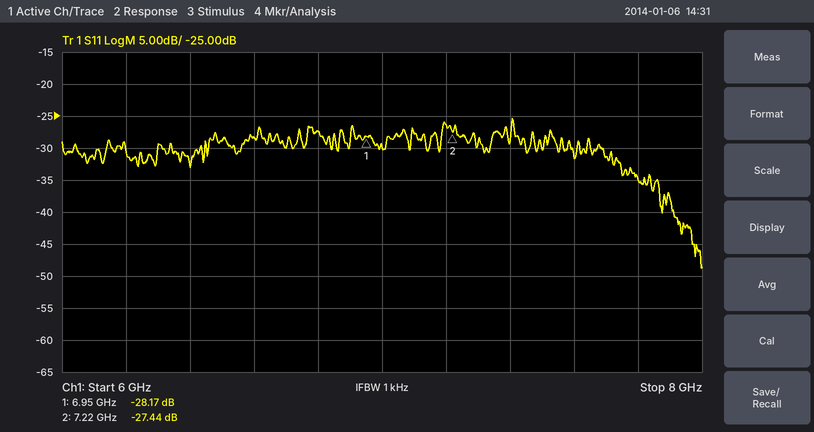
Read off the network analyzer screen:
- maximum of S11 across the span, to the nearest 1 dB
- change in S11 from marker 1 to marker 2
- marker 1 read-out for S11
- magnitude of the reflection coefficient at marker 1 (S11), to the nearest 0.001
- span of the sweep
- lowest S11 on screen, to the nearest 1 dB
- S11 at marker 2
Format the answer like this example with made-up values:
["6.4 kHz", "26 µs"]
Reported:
["-25 dB", "0.73 dB", "-28.17 dB", "0.039", "2 GHz", "-49 dB", "-27.44 dB"]
